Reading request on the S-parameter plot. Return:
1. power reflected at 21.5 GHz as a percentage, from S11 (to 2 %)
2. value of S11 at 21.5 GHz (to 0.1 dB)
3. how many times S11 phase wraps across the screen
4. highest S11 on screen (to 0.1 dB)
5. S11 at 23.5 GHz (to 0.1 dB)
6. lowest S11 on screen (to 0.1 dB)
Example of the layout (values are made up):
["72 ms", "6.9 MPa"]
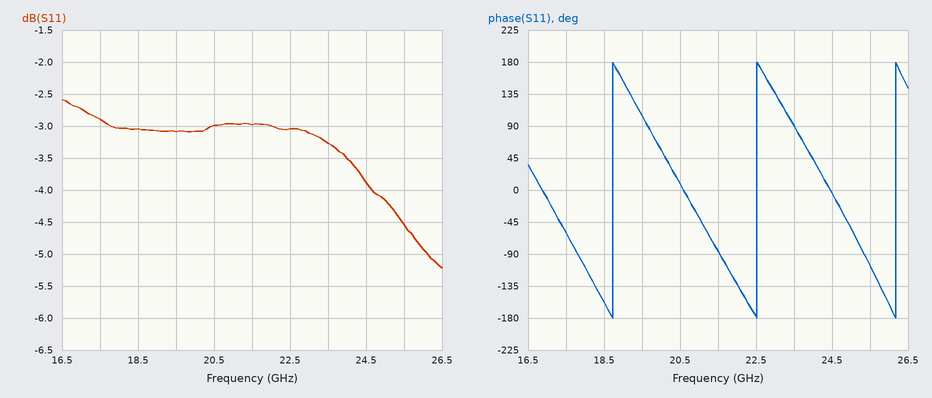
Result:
["50 %", "-3.0 dB", "3", "-2.6 dB", "-3.3 dB", "-5.2 dB"]
